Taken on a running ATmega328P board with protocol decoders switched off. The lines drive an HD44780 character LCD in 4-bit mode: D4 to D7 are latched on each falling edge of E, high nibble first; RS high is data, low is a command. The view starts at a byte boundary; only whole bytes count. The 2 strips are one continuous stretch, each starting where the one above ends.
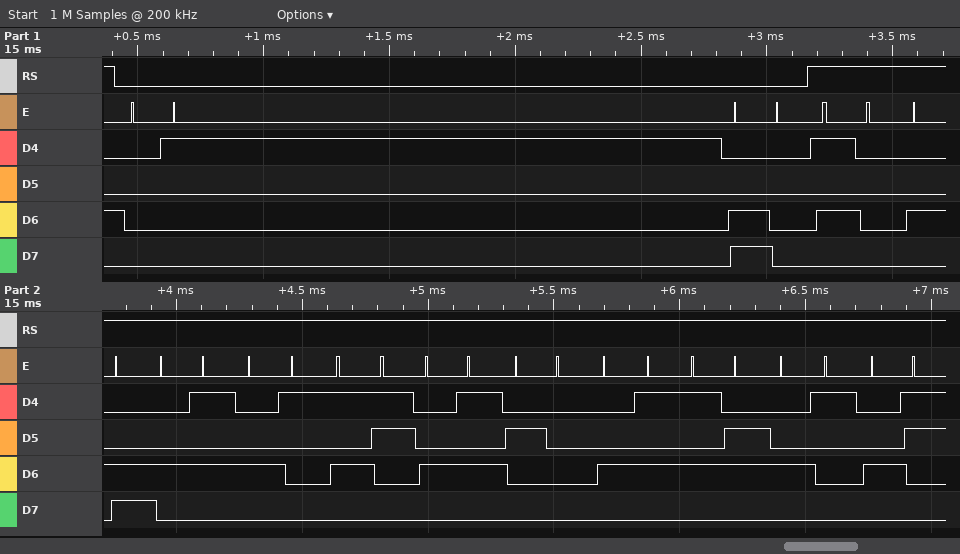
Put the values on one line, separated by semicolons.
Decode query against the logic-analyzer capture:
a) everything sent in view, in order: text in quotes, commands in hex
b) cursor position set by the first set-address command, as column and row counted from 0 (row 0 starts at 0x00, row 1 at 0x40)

0x01 0xC0 "PLEASE EVAC"; column 0, row 1
